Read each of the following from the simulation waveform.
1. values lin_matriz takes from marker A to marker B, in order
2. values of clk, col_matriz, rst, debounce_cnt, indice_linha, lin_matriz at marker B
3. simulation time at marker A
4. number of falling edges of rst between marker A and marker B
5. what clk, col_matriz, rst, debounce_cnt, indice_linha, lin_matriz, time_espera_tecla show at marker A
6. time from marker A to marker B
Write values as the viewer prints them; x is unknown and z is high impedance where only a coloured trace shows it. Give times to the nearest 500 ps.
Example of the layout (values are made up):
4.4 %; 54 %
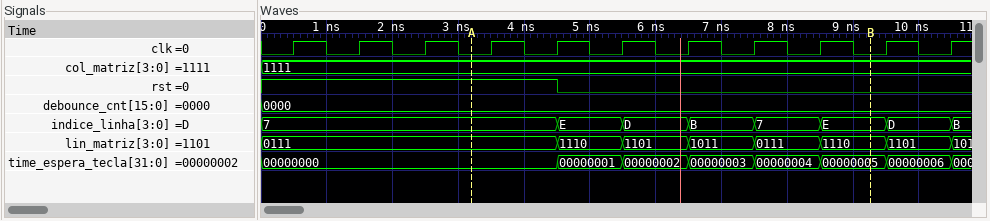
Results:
0111, 1110, 1101, 1011, 0111, 1110; clk=0, col_matriz=1111, rst=0, debounce_cnt=0000, indice_linha=E, lin_matriz=1110; 3000 ps; 1; clk=0, col_matriz=1111, rst=1, debounce_cnt=0000, indice_linha=7, lin_matriz=0111, time_espera_tecla=00000000; 6000 ps
